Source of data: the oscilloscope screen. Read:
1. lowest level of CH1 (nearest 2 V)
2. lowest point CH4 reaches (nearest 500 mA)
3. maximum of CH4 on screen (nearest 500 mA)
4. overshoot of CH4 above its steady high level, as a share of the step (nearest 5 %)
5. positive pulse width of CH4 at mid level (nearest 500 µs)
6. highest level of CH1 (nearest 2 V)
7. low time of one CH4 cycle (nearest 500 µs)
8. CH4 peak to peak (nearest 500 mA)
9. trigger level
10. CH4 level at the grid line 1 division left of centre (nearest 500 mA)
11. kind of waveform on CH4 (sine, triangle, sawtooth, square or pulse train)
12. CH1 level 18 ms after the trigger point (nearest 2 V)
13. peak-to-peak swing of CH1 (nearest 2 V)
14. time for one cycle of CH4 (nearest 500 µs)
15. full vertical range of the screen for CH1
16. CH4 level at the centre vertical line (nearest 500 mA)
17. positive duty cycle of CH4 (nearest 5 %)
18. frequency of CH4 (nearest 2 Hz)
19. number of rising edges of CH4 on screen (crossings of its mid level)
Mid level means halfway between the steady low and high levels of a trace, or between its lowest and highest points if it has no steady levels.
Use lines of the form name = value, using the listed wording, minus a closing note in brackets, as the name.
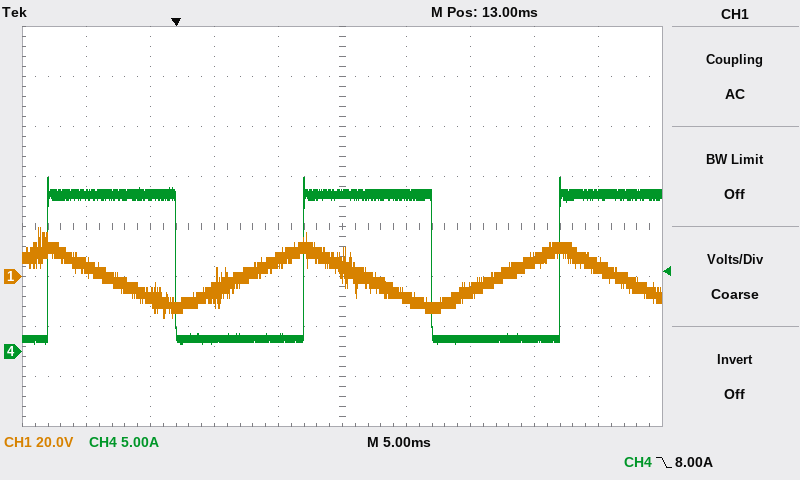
lowest level of CH1 = -16 V
lowest point CH4 reaches = 1.0 A
maximum of CH4 on screen = 17.5 A
overshoot of CH4 above its steady high level, as a share of the step = 10 %
positive pulse width of CH4 at mid level = 10.0 ms
highest level of CH1 = 20 V
low time of one CH4 cycle = 10.0 ms
CH4 peak to peak = 16.5 A
trigger level = 8.00 A
CH4 level at the grid line 1 division left of centre = 1.5 A
kind of waveform on CH4 = square
CH1 level 18 ms after the trigger point = -8 V
peak-to-peak swing of CH1 = 36 V
time for one cycle of CH4 = 20.0 ms
full vertical range of the screen for CH1 = 160 V
CH4 level at the centre vertical line = 16.0 A
positive duty cycle of CH4 = 50 %
frequency of CH4 = 50 Hz
number of rising edges of CH4 on screen = 3
